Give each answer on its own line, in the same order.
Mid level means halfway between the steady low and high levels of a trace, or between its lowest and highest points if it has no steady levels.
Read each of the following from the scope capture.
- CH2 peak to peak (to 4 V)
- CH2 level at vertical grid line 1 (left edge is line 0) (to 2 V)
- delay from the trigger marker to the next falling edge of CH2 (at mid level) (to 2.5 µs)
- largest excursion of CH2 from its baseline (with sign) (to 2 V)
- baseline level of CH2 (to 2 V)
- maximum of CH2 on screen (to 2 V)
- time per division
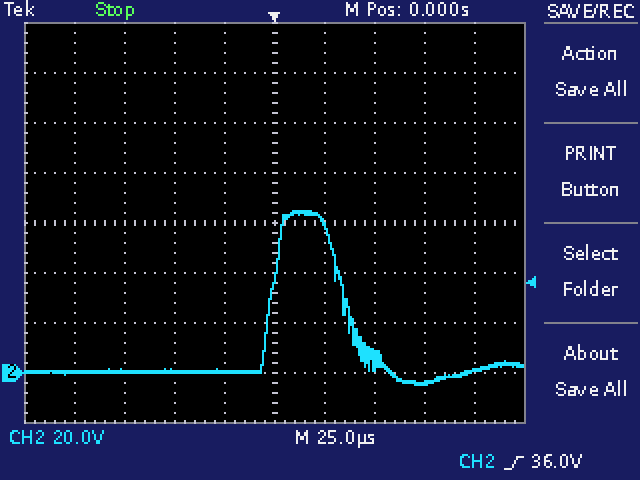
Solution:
68 V
0 V
35.0 µs
+64 V
0 V
64 V
25 µs
